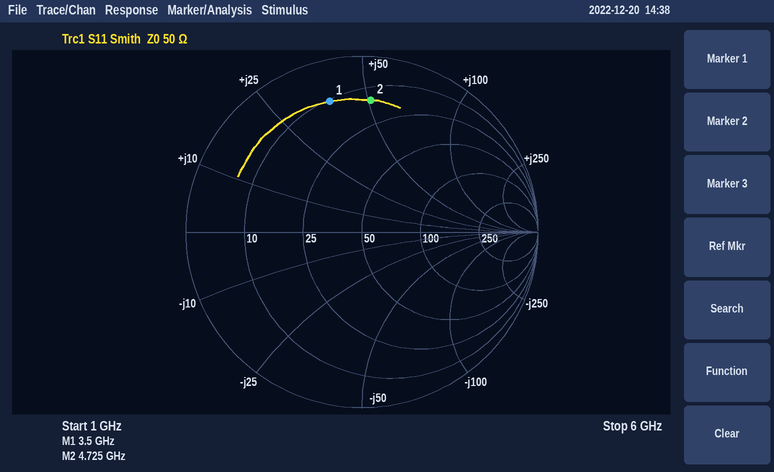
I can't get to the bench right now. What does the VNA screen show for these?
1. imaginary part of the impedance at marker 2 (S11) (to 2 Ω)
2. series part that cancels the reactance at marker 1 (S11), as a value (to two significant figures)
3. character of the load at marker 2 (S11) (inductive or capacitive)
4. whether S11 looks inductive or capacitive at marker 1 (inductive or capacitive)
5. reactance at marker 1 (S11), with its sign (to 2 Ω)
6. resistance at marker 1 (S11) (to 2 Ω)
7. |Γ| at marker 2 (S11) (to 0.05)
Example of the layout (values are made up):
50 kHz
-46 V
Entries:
+52 Ω
1.2 pF
inductive
inductive
+38 Ω
10 Ω
0.75
